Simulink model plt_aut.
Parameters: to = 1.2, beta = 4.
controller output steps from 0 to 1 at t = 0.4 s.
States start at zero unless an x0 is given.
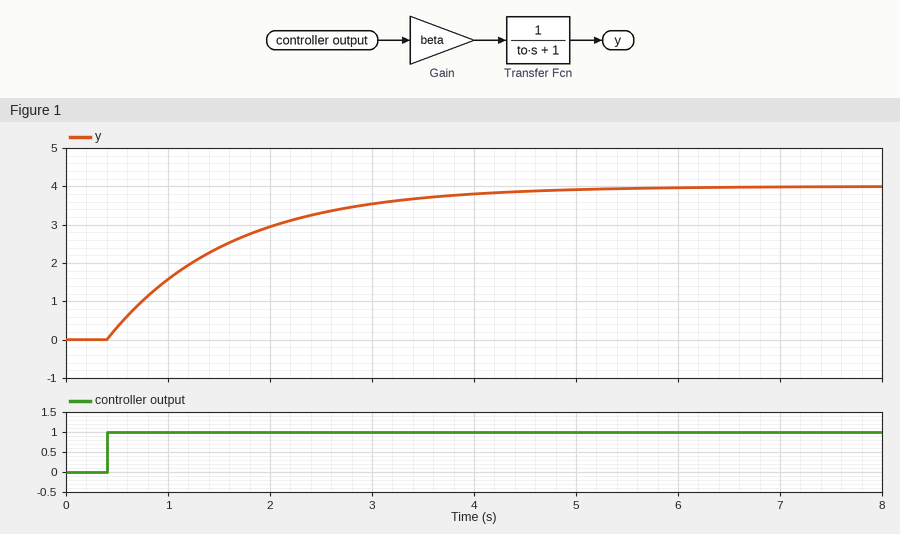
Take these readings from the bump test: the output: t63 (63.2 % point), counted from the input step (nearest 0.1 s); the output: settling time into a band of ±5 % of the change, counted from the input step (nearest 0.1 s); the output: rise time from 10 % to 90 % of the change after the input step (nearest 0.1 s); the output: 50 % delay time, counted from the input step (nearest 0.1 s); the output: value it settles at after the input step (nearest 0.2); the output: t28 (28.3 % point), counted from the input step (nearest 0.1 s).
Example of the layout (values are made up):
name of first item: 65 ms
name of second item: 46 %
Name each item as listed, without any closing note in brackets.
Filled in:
the output: t63 (63.2 % point), counted from the input step: 1.2 s
the output: settling time into a band of ±5 % of the change, counted from the input step: 3.6 s
the output: rise time from 10 % to 90 % of the change after the input step: 2.6 s
the output: 50 % delay time, counted from the input step: 0.8 s
the output: value it settles at after the input step: 4.0
the output: t28 (28.3 % point), counted from the input step: 0.4 s
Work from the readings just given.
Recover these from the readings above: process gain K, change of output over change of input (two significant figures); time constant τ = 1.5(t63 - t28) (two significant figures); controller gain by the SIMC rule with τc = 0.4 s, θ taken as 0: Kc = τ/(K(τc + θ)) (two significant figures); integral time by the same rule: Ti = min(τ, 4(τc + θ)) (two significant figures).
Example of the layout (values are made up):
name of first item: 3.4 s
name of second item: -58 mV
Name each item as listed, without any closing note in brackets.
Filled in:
process gain K, change of output over change of input: 4.0
time constant τ = 1.5(t63 - t28): 1.2 s
controller gain by the SIMC rule with τc = 0.4 s, θ taken as 0: Kc = τ/(K(τc + θ)): 0.75
integral time by the same rule: Ti = min(τ, 4(τc + θ)): 1.2 s
